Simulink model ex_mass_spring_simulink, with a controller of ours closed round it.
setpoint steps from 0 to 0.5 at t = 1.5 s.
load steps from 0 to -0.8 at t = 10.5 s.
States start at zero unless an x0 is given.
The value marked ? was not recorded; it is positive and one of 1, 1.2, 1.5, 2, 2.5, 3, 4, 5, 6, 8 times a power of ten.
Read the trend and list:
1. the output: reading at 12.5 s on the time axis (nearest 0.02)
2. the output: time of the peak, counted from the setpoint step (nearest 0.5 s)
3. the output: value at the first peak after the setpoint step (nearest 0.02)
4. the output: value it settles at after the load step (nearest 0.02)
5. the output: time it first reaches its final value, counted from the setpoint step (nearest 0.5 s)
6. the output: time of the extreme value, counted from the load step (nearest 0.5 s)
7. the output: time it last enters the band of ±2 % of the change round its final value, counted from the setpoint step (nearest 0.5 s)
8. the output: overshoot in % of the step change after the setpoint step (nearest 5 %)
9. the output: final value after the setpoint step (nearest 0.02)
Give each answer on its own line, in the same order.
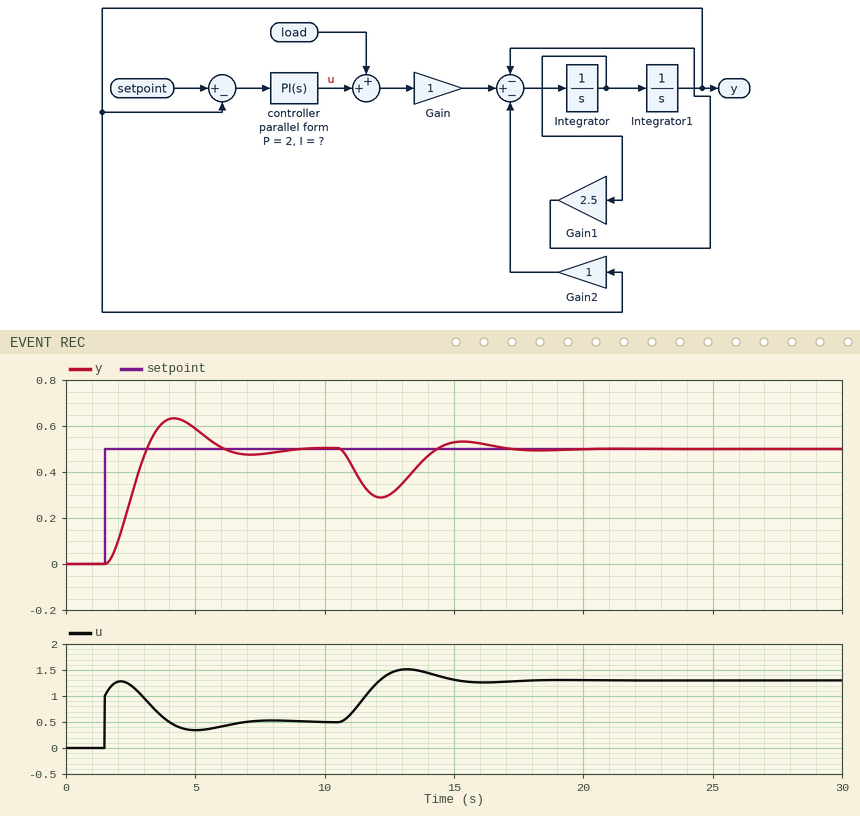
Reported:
0.30
2.5 s
0.64
0.50
1.5 s
1.5 s
7.0 s
25 %
0.50
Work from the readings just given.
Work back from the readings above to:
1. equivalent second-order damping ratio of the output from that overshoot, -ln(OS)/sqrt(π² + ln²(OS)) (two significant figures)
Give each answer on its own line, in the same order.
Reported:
0.40
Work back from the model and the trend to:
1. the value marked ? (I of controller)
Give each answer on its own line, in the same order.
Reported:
2
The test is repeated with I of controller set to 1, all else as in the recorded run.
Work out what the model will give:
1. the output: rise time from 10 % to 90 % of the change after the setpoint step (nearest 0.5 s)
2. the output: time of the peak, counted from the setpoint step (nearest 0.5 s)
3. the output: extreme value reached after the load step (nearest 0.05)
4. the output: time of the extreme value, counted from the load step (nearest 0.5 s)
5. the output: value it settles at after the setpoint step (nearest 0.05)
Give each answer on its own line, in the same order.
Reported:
1.5 s
3.0 s
0.25
2.0 s
0.50
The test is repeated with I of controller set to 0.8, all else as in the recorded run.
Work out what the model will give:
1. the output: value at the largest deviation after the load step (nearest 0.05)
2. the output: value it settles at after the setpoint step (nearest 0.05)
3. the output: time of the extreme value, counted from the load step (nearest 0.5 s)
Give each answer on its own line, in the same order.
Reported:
0.25
0.50
2.0 s
